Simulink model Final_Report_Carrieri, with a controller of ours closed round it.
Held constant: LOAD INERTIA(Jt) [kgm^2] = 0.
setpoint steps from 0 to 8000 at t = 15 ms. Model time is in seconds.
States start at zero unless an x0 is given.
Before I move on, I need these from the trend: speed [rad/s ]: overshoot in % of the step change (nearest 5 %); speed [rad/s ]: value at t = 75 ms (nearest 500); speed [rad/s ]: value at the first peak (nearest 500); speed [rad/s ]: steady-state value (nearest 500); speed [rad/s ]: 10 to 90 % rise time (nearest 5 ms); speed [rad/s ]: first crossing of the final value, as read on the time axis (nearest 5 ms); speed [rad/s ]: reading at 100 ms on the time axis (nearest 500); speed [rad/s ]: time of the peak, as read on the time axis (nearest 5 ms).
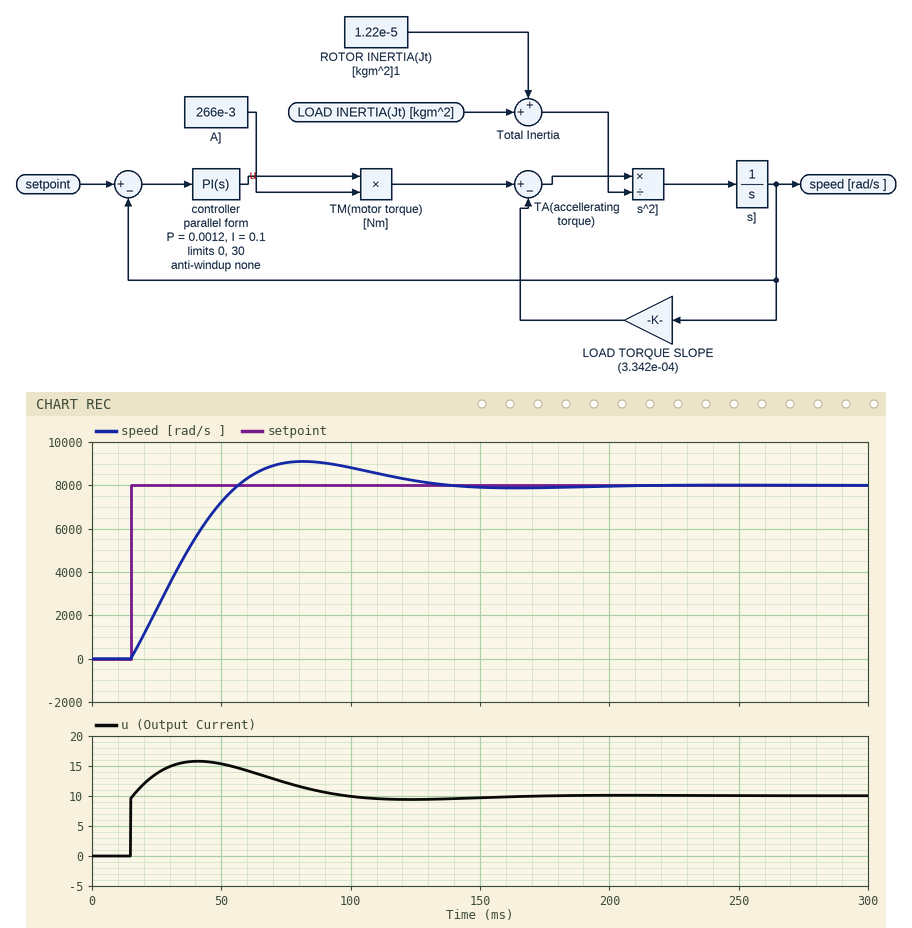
15 %
9000
9000
8000
30 ms
55 ms
9000
80 ms
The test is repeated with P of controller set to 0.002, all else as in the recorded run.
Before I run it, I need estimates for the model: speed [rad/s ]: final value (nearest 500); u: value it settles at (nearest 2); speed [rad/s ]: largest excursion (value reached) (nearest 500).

8000
10
8500
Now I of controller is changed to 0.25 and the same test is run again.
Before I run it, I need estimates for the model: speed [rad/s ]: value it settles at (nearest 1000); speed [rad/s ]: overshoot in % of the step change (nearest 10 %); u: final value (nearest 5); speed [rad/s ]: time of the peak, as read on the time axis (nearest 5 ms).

8000
30 %
10
55 ms
